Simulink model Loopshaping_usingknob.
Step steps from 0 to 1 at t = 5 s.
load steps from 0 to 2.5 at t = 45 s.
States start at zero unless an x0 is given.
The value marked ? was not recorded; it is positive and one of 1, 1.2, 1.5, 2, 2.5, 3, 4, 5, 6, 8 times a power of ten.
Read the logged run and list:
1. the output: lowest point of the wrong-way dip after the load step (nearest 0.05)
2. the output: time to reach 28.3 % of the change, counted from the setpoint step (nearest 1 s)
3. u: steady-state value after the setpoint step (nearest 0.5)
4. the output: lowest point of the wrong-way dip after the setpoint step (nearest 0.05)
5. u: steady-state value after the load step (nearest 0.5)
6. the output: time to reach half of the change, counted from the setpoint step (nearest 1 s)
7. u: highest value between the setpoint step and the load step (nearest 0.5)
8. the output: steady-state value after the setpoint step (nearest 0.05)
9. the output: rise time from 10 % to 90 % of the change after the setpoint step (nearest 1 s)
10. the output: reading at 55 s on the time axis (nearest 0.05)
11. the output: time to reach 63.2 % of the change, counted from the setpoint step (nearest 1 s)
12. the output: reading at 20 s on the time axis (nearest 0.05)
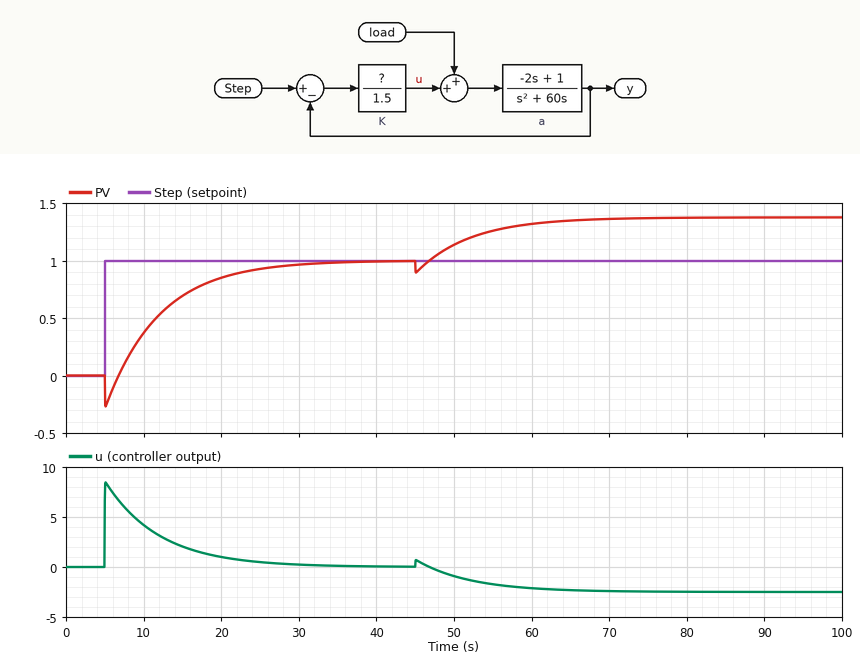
0.90
4 s
0.0
-0.25
-2.5
7 s
8.5
1.00
15 s
1.25
9 s
0.85
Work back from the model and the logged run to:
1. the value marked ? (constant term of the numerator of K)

10
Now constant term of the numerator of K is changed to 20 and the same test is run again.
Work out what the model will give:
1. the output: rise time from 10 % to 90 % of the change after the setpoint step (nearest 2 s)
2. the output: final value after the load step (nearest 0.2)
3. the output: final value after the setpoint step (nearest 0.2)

6 s
1.2
1.0
